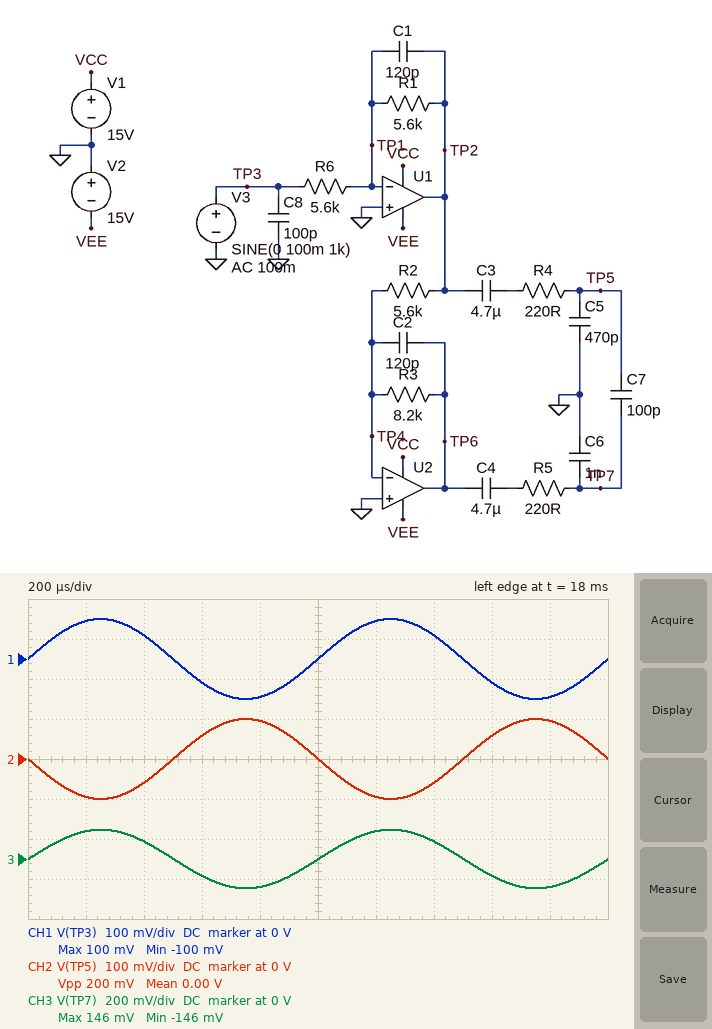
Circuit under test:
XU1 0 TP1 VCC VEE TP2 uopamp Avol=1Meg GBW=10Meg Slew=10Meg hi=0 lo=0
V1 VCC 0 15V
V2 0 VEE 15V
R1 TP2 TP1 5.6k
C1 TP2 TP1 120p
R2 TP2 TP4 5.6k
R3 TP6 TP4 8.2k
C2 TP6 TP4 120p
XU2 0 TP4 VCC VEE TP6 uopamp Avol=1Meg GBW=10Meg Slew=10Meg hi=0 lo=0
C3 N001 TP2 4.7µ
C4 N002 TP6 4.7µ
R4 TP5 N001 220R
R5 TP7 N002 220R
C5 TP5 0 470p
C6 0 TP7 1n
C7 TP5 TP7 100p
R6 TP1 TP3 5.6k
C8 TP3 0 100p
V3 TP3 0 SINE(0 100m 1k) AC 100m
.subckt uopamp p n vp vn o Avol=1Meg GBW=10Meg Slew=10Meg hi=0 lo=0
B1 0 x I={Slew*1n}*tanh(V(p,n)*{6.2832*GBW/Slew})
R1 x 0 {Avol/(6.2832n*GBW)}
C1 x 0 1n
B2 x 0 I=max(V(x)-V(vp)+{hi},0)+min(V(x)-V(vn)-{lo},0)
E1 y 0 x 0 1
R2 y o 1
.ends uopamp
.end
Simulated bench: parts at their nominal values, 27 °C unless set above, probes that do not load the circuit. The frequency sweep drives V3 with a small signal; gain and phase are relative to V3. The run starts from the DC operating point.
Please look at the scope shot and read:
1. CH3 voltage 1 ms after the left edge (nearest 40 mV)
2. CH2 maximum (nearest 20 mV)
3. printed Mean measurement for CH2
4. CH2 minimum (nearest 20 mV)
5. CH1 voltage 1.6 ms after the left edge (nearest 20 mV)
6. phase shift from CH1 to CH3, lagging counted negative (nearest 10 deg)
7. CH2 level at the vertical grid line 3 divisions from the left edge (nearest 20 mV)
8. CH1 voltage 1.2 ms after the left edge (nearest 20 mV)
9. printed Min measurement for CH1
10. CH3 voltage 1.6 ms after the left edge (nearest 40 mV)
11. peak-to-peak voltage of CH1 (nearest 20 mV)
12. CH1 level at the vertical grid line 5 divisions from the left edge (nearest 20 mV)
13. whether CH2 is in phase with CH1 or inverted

0 V
100 mV
0.00 V
-100 mV
-60 mV
0 deg
60 mV
100 mV
-100 mV
-80 mV
200 mV
0 V
inverted
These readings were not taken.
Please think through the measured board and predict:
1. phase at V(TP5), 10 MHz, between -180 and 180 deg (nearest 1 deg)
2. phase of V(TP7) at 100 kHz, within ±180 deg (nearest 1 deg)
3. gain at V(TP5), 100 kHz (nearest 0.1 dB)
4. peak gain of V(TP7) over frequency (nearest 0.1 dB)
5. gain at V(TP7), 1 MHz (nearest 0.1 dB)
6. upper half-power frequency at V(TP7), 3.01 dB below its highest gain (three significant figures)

-36 deg
-66 deg
-0.9 dB
3.3 dB
-28.2 dB
118 kHz
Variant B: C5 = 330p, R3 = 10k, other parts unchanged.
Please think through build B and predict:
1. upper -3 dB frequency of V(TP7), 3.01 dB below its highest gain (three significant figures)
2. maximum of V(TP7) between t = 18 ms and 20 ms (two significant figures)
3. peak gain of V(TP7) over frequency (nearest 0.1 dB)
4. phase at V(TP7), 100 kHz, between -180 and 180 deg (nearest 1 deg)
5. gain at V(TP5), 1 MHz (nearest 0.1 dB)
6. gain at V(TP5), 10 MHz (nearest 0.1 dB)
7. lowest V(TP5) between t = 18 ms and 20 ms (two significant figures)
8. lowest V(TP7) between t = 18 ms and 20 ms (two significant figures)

104 kHz
180 mV
5.0 dB
-71 deg
-14.4 dB
-51.0 dB
-100 mV
-180 mV
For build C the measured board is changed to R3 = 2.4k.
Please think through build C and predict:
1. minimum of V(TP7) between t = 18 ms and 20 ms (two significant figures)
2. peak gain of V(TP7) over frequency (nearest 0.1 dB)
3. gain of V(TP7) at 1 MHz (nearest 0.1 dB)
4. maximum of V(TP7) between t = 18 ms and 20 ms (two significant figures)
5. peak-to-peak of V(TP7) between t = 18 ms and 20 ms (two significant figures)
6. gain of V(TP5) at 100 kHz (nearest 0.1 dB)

-43 mV
-7.4 dB
-29.5 dB
43 mV
86 mV
-0.8 dB
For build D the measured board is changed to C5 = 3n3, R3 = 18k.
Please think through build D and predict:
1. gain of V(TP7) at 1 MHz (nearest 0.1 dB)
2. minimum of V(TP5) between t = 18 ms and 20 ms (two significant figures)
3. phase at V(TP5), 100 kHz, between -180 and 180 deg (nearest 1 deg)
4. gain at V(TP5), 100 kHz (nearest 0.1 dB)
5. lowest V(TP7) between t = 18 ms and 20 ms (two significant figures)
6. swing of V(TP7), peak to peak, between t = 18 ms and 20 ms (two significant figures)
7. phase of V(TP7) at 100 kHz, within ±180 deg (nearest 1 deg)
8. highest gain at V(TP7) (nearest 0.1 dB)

-30.6 dB
-100 mV
130 deg
-1.8 dB
-320 mV
640 mV
-88 deg
10.1 dB
